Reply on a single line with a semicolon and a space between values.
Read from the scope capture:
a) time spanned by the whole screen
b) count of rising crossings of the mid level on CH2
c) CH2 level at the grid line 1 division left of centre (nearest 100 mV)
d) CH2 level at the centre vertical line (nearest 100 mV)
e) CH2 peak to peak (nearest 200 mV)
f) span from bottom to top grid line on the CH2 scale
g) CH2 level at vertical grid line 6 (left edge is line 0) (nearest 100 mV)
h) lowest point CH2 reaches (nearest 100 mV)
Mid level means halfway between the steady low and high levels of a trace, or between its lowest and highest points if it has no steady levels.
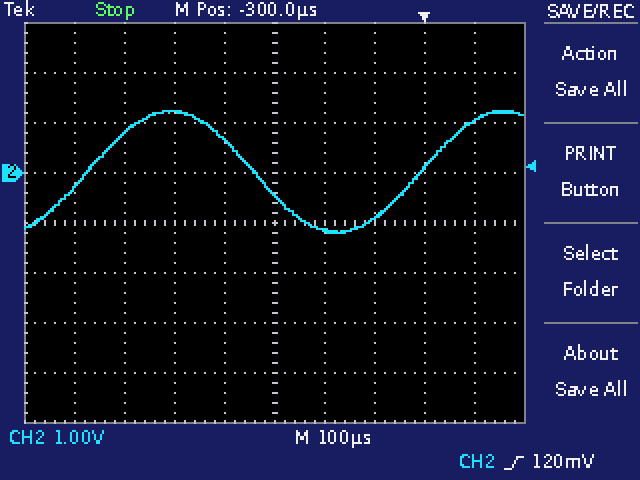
1 ms; 2; 700 mV; -400 mV; 2.4 V; 8 V; -1.2 V; -1.2 V
